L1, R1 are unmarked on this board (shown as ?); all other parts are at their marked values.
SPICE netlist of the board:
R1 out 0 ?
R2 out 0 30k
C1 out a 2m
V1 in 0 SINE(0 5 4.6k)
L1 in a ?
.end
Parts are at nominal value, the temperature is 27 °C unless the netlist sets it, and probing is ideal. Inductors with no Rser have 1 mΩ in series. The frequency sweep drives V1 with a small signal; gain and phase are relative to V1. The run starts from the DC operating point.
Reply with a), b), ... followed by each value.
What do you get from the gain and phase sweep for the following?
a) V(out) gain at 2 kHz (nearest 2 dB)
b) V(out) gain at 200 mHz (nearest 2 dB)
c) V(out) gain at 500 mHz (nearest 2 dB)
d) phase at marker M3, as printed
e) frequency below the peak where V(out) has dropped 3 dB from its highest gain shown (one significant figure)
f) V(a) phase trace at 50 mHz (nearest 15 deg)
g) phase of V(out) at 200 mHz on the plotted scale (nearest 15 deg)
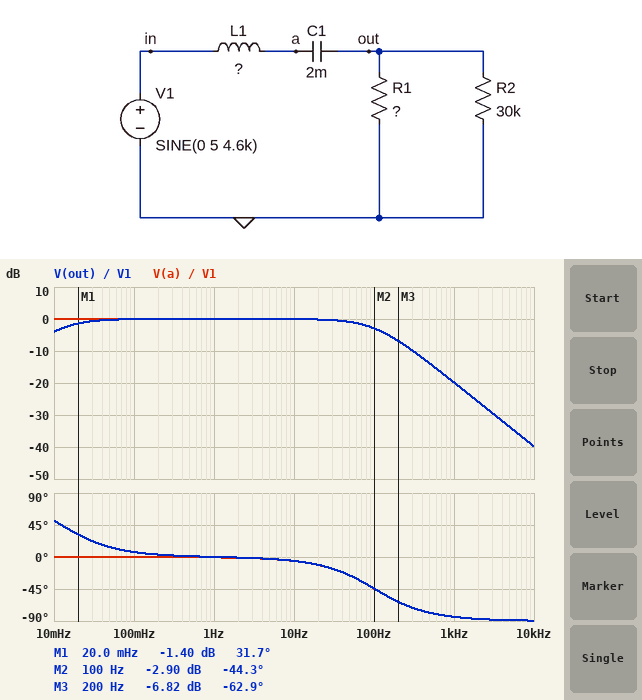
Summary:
a) -26 dB
b) 0 dB
c) 0 dB
d) -62.9 deg
e) 10 mHz
f) 0 deg
g) 0 deg
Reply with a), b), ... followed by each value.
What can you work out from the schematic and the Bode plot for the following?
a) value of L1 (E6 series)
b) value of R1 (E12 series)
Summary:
a) 10 H
b) 8.2 kΩ
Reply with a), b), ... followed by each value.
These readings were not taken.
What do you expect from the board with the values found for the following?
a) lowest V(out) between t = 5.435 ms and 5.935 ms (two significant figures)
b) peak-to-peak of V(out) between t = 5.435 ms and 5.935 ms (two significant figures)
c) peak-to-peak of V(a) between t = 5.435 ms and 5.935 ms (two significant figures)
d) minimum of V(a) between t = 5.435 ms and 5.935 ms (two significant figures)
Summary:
a) -110 mV
b) 220 mV
c) 220 mV
d) -110 mV
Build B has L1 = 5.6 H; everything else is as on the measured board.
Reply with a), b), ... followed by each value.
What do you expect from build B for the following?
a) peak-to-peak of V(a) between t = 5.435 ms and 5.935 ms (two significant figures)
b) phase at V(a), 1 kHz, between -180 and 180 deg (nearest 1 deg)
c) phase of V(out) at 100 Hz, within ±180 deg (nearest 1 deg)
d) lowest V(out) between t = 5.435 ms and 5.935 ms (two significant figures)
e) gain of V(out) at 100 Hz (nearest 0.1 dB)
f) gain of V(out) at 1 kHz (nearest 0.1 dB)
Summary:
a) 400 mV
b) -80 deg
c) -29 deg
d) -200 mV
e) -1.1 dB
f) -14.9 dB
